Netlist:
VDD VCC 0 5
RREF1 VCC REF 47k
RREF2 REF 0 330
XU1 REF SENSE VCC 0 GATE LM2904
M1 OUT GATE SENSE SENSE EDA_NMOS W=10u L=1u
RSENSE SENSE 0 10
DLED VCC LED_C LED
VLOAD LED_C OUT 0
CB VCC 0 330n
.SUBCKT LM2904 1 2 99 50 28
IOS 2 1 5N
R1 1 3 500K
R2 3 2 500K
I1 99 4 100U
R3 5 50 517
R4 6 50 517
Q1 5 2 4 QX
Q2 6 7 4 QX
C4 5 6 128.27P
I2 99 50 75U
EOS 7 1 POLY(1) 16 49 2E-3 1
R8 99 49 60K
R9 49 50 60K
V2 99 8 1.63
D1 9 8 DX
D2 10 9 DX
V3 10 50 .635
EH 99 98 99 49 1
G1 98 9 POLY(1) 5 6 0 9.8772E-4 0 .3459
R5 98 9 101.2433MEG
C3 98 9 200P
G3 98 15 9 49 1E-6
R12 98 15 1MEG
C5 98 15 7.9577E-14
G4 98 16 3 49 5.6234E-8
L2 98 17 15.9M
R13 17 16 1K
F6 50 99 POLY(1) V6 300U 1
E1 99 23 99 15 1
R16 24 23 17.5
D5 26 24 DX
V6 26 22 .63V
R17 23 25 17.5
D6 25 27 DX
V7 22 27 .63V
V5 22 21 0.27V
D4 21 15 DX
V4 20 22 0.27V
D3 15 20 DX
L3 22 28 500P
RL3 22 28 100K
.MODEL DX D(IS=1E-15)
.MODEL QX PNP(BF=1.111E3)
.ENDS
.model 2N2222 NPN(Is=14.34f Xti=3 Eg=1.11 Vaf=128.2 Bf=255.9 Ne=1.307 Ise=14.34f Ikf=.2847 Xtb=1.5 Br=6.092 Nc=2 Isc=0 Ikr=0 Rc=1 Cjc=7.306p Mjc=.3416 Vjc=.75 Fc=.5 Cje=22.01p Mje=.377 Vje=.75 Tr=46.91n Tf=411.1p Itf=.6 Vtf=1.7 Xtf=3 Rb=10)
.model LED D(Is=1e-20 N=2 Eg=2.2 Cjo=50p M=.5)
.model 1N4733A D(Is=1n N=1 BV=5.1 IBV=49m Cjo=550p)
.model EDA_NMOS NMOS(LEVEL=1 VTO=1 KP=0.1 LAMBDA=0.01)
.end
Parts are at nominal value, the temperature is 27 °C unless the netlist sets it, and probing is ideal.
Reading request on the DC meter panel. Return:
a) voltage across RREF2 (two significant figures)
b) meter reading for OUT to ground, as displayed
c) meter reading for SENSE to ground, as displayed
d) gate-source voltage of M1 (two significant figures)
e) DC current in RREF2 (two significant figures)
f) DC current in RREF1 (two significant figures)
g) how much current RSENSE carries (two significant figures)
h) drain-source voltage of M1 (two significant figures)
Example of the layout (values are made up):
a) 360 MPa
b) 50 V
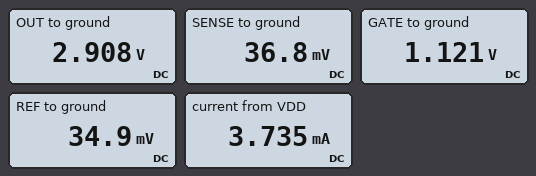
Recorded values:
a) 35 mV
b) 2.908 V
c) 36.8 mV
d) 1.1 V
e) 110 µA
f) 110 µA
g) 3.7 mA
h) 2.9 V
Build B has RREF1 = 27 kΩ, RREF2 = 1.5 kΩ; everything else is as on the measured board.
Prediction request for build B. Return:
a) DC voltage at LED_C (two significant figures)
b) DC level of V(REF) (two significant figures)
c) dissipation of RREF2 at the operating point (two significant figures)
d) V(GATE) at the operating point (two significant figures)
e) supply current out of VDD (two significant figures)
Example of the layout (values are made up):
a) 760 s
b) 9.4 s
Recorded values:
a) 2.8 V
b) 260 mV
c) 46 µW
d) 1.5 V
e) 27 mA
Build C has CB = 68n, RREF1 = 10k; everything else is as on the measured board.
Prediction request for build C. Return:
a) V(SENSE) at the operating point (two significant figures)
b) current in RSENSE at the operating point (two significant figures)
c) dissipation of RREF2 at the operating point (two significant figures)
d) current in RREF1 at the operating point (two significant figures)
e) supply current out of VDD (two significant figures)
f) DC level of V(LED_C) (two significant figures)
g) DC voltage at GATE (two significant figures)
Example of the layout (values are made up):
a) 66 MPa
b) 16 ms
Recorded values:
a) 160 mV
b) 16 mA
c) 77 µW
d) 480 µA
e) 17 mA
f) 2.8 V
g) 1.3 V
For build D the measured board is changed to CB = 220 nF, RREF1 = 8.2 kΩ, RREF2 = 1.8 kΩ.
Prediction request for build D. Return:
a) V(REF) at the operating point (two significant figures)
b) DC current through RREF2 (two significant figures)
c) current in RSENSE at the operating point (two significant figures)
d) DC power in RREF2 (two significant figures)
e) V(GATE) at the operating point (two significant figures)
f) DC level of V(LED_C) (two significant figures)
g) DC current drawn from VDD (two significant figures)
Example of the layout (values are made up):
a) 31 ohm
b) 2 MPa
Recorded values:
a) 900 mV
b) 500 µA
c) 90 mA
d) 450 µW
e) 2.3 V
f) 2.7 V
g) 91 mA
